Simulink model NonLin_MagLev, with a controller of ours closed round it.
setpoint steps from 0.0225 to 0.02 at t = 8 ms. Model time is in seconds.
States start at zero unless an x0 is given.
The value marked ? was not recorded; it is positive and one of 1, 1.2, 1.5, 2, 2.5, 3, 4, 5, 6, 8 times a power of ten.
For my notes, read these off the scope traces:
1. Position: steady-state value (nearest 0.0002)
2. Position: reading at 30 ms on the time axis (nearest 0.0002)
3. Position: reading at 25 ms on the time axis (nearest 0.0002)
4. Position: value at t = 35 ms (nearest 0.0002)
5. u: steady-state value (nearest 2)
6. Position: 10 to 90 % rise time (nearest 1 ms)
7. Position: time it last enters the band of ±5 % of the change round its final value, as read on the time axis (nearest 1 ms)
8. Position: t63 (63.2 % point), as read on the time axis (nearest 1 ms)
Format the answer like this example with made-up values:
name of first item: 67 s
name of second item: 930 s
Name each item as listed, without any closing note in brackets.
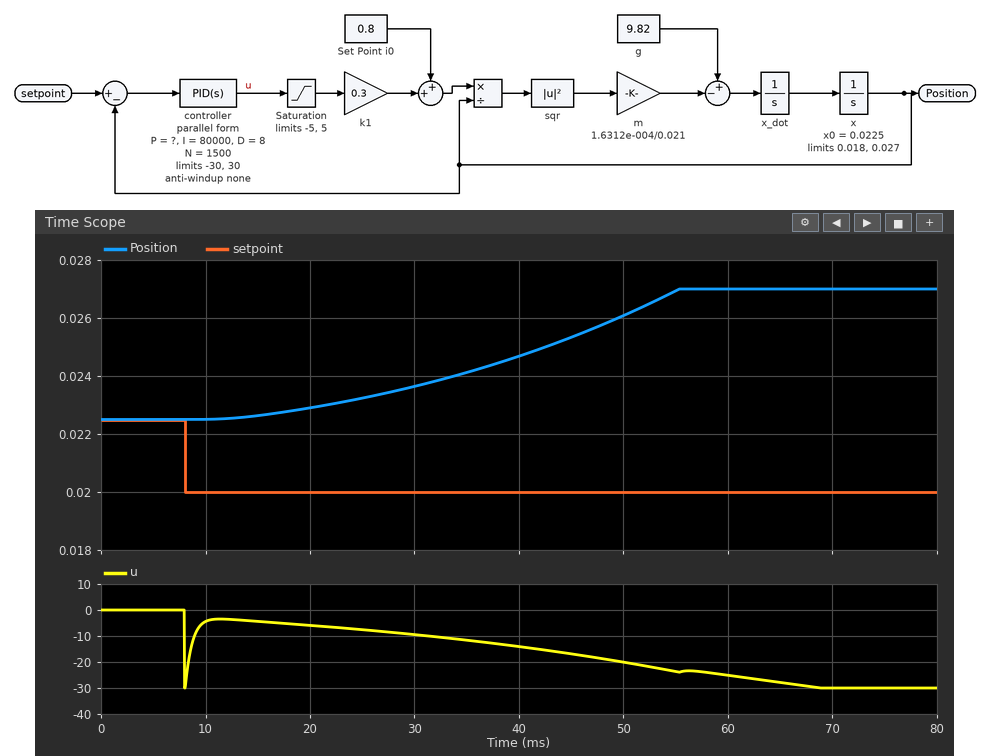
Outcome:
Position: steady-state value: 0.0270
Position: reading at 30 ms on the time axis: 0.0236
Position: reading at 25 ms on the time axis: 0.0232
Position: value at t = 35 ms: 0.0242
u: steady-state value: -30
Position: 10 to 90 % rise time: 32 ms
Position: time it last enters the band of ±5 % of the change round its final value, as read on the time axis: 54 ms
Position: t63 (63.2 % point), as read on the time axis: 45 ms
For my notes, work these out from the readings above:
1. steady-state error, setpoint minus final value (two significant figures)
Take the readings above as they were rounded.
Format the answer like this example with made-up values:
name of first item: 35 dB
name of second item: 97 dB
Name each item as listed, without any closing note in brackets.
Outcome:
steady-state error, setpoint minus final value: -0.0070
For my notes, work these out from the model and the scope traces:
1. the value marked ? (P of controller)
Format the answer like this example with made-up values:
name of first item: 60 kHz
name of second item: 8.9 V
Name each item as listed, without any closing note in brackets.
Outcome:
the value marked ?: 1000
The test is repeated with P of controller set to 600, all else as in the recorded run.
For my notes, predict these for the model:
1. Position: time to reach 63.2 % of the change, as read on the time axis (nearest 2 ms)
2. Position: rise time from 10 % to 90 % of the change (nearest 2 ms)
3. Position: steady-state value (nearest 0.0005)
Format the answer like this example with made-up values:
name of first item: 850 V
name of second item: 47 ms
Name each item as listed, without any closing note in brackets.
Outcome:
Position: time to reach 63.2 % of the change, as read on the time axis: 40 ms
Position: rise time from 10 % to 90 % of the change: 28 ms
Position: steady-state value: 0.0270
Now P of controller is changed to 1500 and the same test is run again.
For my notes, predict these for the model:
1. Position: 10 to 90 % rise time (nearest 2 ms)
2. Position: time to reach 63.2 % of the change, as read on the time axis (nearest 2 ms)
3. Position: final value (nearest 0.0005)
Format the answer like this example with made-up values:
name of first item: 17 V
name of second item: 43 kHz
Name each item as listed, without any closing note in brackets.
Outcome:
Position: 10 to 90 % rise time: 36 ms
Position: time to reach 63.2 % of the change, as read on the time axis: 54 ms
Position: final value: 0.0270
